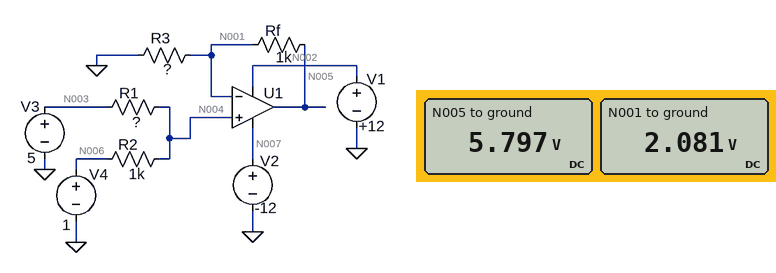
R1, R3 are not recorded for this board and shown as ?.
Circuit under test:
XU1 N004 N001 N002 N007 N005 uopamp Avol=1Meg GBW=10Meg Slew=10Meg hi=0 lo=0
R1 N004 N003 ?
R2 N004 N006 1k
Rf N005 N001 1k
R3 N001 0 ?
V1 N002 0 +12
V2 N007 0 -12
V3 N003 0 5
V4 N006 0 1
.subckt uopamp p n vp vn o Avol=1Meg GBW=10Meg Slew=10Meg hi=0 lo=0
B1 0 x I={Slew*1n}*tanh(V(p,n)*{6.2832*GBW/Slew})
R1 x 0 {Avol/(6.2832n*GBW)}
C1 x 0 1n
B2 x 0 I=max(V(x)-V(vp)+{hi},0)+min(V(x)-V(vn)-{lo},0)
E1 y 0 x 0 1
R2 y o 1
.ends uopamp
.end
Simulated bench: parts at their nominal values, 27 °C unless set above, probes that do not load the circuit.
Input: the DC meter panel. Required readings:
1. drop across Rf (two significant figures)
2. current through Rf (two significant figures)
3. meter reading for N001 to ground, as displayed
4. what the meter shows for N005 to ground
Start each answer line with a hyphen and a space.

- 3.7 V
- 3.7 mA
- 2.081 V
- 5.797 V
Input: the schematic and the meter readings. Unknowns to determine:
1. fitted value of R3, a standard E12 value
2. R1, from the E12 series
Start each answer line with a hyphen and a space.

- 560 Ω
- 2.7 kΩ
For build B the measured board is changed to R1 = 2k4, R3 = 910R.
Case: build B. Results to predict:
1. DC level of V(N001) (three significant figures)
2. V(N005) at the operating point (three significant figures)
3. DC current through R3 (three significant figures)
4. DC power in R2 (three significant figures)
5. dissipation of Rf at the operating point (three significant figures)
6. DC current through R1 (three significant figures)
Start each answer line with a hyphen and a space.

- 2.18 V
- 4.57 V
- 2.39 mA
- 1.38 mW
- 5.72 mW
- 1.18 mA
